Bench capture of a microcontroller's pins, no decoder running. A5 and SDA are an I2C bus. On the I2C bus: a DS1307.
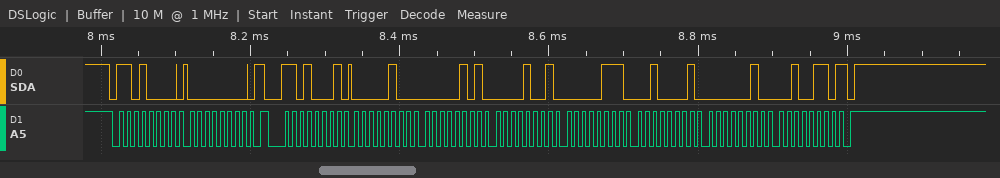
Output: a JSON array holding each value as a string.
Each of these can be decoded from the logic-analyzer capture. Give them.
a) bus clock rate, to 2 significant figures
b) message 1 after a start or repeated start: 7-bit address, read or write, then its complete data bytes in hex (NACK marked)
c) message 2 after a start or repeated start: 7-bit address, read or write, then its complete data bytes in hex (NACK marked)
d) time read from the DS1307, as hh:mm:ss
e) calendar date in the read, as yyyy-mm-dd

["100 kHz", "0x68 write: 00", "0x68 read: 04 05 09 07 21 02 26 NACK", "09:05:04", "2026-02-21"]
